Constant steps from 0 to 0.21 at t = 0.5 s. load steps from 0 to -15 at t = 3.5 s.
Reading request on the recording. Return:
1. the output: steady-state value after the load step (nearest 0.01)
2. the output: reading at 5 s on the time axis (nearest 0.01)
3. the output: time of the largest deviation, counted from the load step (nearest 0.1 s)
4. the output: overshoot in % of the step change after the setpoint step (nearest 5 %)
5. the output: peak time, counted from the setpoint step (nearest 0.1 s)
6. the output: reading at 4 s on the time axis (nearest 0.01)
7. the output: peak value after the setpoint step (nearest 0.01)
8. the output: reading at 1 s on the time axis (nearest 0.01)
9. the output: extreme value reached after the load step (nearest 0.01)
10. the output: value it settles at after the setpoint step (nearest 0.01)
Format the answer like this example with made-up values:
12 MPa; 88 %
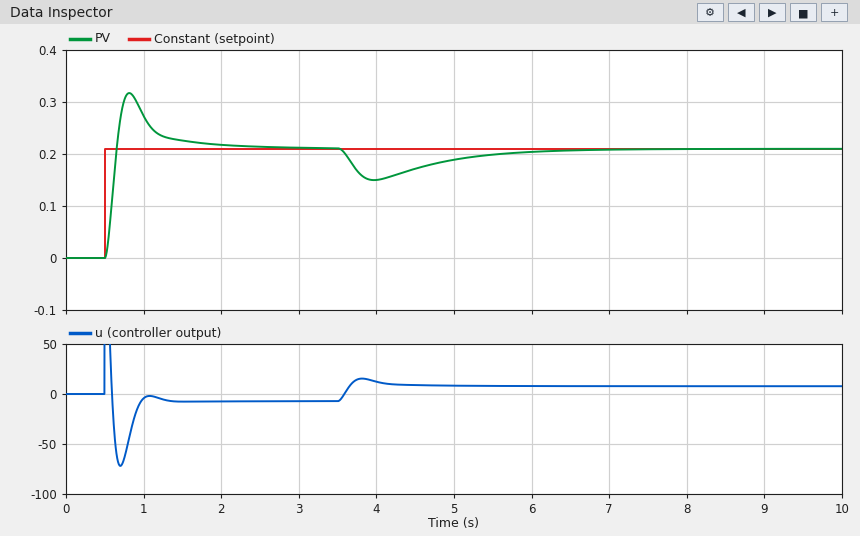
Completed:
0.21; 0.19; 0.5 s; 50 %; 0.3 s; 0.15; 0.32; 0.27; 0.15; 0.21
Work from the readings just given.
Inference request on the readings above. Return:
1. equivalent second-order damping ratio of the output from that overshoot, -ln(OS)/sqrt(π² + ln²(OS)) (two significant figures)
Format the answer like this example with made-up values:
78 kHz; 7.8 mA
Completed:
0.22
